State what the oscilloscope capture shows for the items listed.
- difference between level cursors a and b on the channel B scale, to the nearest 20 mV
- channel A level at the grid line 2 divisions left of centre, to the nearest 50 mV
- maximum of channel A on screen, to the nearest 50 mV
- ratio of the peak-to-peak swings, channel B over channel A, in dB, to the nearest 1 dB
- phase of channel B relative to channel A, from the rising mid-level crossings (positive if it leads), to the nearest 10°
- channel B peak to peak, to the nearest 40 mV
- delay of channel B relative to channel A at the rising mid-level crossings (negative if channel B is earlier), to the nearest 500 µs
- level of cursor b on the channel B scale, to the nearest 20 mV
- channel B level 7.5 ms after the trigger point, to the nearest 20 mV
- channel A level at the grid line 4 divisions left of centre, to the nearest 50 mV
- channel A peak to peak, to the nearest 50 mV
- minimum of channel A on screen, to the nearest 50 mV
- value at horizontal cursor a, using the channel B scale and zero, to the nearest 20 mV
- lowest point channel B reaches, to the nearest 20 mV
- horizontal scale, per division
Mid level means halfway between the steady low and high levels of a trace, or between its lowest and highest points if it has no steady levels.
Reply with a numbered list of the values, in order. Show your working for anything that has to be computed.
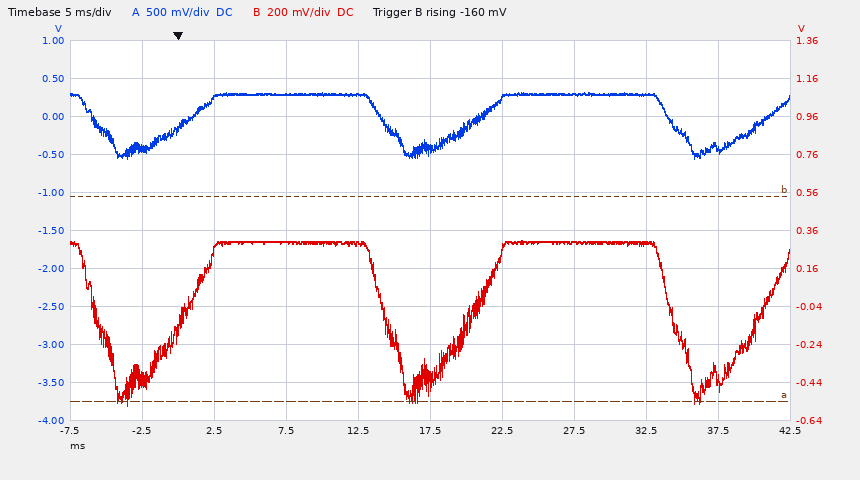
1. 1.08 V
2. 300 mV
3. 300 mV
4. 20 log10(880 mV / 850 mV) ≈ 0 dB
5. 0°
6. 880 mV
7. 0.0 ms
8. 540 mV
9. 300 mV
10. -400 mV
11. 300 mV − (-550 mV) = 850 mV
12. -550 mV
13. -540 mV
14. -560 mV
15. 5 ms
